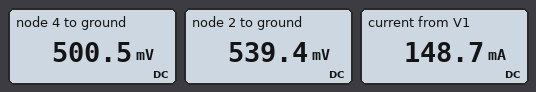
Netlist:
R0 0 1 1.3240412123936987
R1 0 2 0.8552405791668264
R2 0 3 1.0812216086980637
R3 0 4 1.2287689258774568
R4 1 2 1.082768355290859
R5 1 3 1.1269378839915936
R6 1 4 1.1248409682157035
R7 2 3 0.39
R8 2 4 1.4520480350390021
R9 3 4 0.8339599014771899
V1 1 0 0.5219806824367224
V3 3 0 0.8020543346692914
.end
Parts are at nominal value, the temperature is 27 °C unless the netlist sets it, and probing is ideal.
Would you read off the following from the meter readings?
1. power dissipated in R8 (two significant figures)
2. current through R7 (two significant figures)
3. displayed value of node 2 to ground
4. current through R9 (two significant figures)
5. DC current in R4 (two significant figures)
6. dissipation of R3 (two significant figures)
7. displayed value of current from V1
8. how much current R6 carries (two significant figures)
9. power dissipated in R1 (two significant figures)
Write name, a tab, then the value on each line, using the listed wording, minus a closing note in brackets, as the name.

power dissipated in R8	1.0 mW
current through R7	670 mA
displayed value of node 2 to ground	539.4 mV
current through R9	360 mA
DC current in R4	16 mA
dissipation of R3	200 mW
displayed value of current from V1	148.7 mA
how much current R6 carries	19 mA
power dissipated in R1	340 mW
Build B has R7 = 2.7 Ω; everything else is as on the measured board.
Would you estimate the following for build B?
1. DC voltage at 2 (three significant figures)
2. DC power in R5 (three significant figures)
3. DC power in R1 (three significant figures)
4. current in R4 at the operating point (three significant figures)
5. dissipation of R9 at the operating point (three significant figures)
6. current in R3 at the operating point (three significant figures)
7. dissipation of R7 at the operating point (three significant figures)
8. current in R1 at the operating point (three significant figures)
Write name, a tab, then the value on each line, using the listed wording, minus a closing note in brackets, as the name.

DC voltage at 2	349 mV
DC power in R5	69.6 mW
DC power in R1	142 mW
current in R4 at the operating point	160 mA
dissipation of R9 at the operating point	137 mW
current in R3 at the operating point	378 mA
dissipation of R7 at the operating point	76.2 mW
current in R1 at the operating point	408 mA
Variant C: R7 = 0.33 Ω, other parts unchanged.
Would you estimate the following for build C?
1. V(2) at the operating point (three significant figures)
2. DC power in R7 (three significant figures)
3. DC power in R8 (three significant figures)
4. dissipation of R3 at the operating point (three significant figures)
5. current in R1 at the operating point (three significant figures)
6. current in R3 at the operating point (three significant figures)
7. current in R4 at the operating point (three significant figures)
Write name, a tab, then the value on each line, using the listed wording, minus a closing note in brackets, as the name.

V(2) at the operating point	561 mV
DC power in R7	176 mW
DC power in R8	2.18 mW
dissipation of R3 at the operating point	207 mW
current in R1 at the operating point	656 mA
current in R3 at the operating point	411 mA
current in R4 at the operating point	36.0 mA
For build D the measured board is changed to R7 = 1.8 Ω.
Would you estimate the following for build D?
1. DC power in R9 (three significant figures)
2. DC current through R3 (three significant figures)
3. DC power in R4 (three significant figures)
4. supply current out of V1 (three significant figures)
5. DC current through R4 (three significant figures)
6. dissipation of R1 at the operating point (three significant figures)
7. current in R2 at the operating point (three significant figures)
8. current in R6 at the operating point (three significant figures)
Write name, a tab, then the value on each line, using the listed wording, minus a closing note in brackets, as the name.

DC power in R9	133 mW
DC current through R3	382 mA
DC power in R4	20.0 mW
supply current out of V1	329 mA
DC current through R4	136 mA
dissipation of R1 at the operating point	164 mW
current in R2 at the operating point	742 mA
current in R6 at the operating point	47.1 mA
